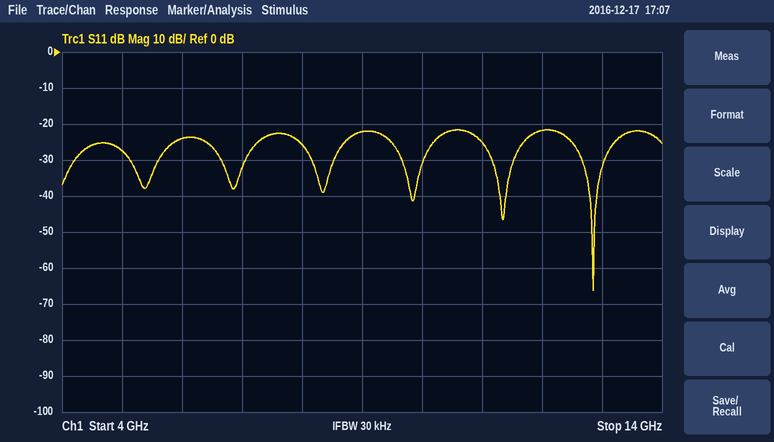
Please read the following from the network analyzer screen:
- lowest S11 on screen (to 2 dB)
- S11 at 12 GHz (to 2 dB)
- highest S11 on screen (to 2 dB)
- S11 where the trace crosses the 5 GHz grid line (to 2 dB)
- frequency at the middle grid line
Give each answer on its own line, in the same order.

-66 dB
-22 dB
-22 dB
-28 dB
9 GHz
